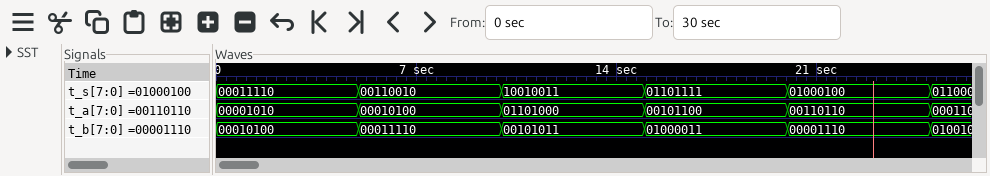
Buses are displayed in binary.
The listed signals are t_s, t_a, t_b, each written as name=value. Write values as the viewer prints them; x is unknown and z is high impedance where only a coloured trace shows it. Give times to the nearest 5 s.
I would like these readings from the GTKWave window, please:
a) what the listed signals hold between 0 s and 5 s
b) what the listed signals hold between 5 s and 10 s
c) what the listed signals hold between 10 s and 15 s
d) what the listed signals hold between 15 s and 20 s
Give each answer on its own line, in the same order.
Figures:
t_s=00011110, t_a=00001010, t_b=00010100
t_s=00110010, t_a=00010100, t_b=00011110
t_s=10010011, t_a=01101000, t_b=00101011
t_s=01101111, t_a=00101100, t_b=01000011
